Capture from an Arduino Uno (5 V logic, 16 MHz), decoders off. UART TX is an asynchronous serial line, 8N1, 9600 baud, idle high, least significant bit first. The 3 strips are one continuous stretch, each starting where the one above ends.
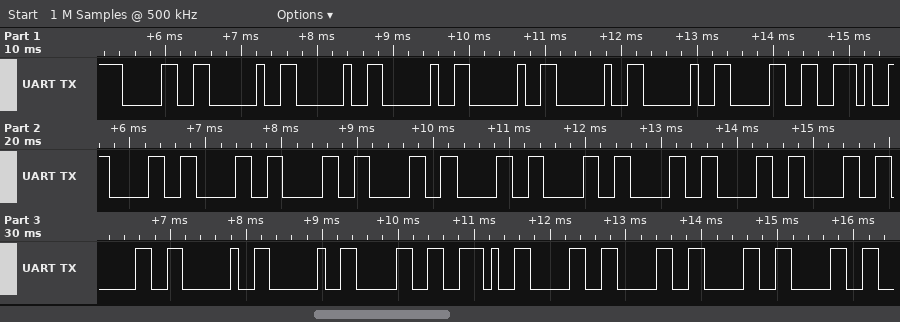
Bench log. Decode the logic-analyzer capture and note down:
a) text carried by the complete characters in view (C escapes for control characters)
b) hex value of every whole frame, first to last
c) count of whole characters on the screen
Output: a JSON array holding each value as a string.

["\"0      0.0000000000  0.0000\"", "30 20 20 20 20 20 20 30 2E 30 30 30 30 30 30 30 30 30 30 20 20 30 2E 30 30 30 30", "27"]
